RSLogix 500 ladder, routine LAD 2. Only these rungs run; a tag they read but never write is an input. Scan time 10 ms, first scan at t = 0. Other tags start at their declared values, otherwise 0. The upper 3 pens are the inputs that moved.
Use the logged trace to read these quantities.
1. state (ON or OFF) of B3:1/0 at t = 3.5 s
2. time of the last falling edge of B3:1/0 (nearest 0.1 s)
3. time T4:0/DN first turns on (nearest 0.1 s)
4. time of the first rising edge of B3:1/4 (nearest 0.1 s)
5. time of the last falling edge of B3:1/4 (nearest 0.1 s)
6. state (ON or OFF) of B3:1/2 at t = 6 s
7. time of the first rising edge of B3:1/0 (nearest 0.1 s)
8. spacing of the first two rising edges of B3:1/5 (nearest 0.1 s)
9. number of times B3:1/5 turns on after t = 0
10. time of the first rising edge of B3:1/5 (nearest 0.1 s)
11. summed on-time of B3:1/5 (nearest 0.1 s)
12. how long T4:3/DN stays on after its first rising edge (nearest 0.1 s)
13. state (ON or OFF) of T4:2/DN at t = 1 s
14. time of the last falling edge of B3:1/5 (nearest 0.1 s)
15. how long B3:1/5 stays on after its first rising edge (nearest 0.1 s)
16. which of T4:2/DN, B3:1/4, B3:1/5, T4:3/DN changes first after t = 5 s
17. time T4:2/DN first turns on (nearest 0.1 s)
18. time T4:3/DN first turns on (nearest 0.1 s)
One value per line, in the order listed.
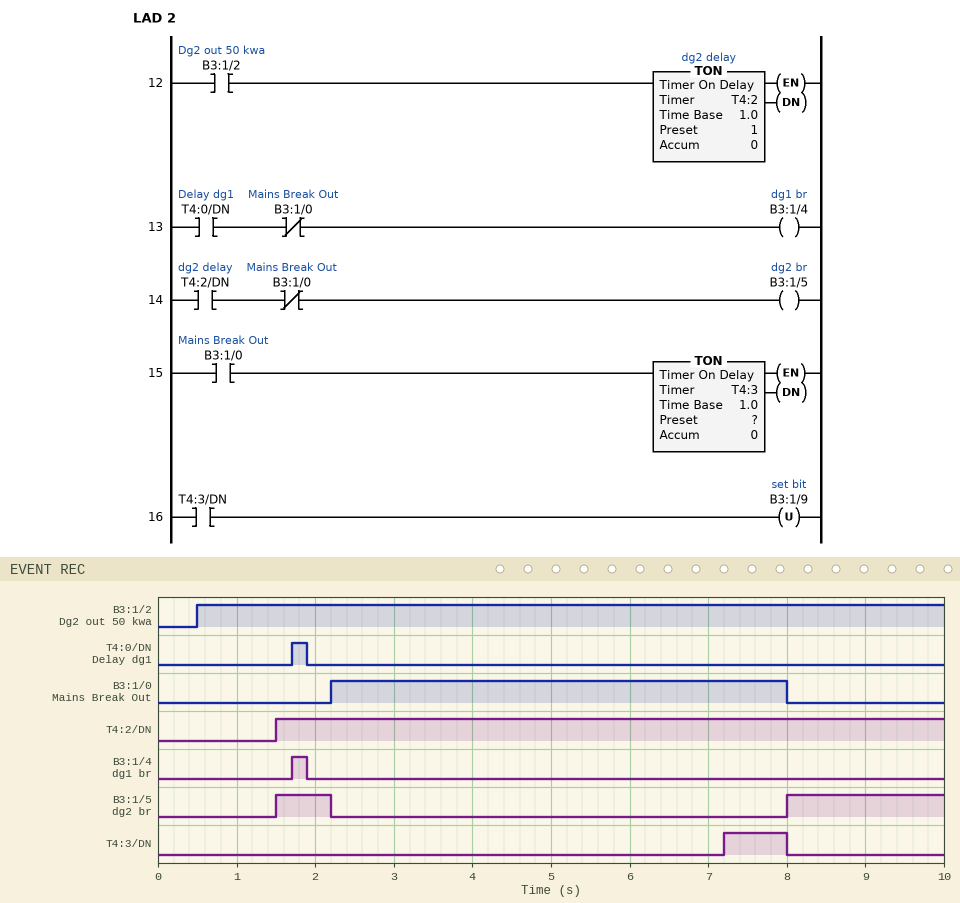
ON
8.0 s
1.7 s
1.7 s
1.9 s
ON
2.2 s
6.5 s
2
1.5 s
2.7 s
0.8 s
OFF
2.2 s
0.7 s
T4:3/DN
1.5 s
7.2 s
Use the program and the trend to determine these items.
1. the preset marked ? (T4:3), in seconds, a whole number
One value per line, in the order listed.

5 s
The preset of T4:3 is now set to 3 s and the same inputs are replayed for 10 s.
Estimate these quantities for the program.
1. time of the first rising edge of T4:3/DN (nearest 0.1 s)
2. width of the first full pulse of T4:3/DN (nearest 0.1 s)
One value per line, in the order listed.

5.2 s
2.8 s
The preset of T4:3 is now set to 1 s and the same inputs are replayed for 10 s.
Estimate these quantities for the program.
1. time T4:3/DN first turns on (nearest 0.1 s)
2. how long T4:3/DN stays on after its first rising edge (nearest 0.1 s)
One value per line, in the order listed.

3.2 s
4.8 s
